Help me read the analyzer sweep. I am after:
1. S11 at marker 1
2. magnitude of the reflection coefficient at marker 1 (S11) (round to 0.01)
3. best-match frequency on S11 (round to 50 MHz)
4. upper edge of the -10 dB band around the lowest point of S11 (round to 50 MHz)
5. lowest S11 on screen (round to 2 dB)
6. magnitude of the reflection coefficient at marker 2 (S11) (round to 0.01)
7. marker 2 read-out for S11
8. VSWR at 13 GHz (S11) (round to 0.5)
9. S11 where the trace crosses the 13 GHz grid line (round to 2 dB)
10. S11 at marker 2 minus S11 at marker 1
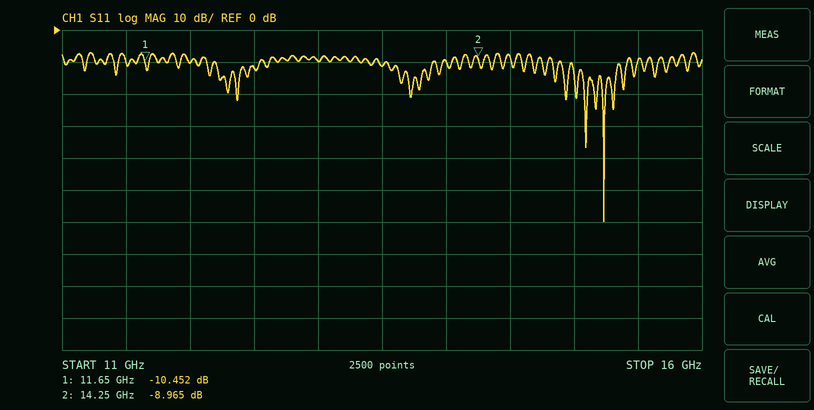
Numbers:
-10.452 dB
0.30
15.25 GHz
15.40 GHz
-60 dB
0.36
-8.965 dB
2.0
-10 dB
1.487 dB
